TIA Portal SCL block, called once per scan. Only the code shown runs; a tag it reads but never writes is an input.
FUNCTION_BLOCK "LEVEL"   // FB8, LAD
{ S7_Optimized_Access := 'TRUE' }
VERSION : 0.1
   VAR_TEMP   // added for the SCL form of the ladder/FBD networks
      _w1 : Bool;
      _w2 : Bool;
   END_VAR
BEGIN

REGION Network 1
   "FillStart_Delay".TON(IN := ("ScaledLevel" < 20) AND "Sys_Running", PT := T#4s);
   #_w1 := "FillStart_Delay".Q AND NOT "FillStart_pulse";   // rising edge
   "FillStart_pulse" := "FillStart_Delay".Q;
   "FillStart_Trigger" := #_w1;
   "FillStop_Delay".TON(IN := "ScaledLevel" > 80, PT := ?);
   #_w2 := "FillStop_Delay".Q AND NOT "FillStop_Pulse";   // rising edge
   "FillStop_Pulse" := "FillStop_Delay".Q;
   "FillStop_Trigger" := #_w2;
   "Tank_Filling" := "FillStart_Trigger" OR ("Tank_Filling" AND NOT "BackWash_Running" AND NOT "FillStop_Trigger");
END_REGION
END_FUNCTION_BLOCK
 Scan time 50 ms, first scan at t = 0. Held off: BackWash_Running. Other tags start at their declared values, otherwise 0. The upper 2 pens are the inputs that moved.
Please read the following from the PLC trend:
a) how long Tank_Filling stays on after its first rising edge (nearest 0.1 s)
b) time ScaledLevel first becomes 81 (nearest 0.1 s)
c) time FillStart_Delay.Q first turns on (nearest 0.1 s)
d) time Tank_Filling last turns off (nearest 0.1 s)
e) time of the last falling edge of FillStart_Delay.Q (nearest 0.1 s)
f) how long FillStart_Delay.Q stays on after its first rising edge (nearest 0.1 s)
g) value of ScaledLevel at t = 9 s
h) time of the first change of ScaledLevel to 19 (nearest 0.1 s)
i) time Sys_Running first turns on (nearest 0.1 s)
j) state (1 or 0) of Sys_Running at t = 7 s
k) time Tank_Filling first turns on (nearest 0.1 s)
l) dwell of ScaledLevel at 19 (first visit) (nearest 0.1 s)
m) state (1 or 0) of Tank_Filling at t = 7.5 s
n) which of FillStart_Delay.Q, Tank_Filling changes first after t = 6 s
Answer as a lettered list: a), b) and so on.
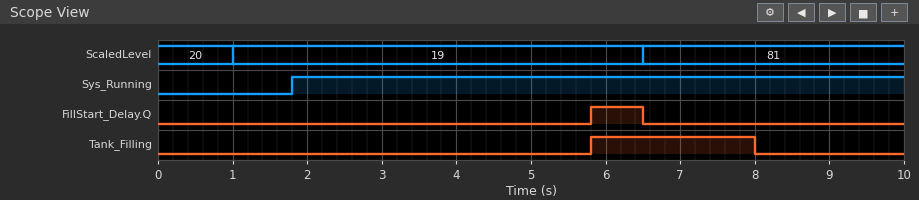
a) 2.2 s
b) 6.5 s
c) 5.8 s
d) 8.0 s
e) 6.5 s
f) 0.7 s
g) 81
h) 1.0 s
i) 1.8 s
j) 1
k) 5.8 s
l) 5.5 s
m) 1
n) FillStart_Delay.Q
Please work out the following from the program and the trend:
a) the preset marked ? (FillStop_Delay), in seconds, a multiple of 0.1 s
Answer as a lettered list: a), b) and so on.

a) 1.5 s
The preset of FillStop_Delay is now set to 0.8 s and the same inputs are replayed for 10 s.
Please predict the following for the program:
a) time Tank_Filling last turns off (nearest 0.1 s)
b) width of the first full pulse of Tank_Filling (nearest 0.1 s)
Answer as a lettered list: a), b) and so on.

a) 7.3 s
b) 1.5 s
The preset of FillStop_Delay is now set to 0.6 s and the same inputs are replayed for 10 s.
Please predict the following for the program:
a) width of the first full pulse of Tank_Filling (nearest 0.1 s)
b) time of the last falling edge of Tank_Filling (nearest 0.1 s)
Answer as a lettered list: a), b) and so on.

a) 1.3 s
b) 7.1 s
